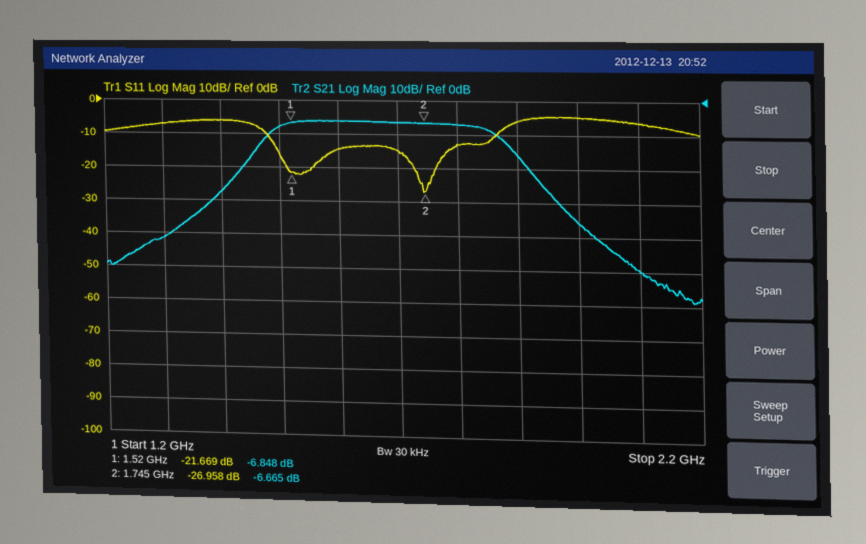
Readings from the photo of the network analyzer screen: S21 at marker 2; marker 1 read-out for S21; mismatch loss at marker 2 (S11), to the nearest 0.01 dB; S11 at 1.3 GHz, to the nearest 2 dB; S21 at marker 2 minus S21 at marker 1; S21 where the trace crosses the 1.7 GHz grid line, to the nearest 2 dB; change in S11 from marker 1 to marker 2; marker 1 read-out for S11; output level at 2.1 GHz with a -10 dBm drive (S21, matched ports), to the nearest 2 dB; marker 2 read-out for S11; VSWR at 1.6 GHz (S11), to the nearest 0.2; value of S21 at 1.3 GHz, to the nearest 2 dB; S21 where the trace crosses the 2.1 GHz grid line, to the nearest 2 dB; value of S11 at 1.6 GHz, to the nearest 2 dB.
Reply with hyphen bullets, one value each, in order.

- -6.665 dB
- -6.848 dB
- 0.01 dB
- -8 dB
- 0.183 dB
- -6 dB
- -5.289 dB
- -21.669 dB
- -60 dBm
- -26.958 dB
- 1.4
- -42 dB
- -50 dB
- -14 dB
